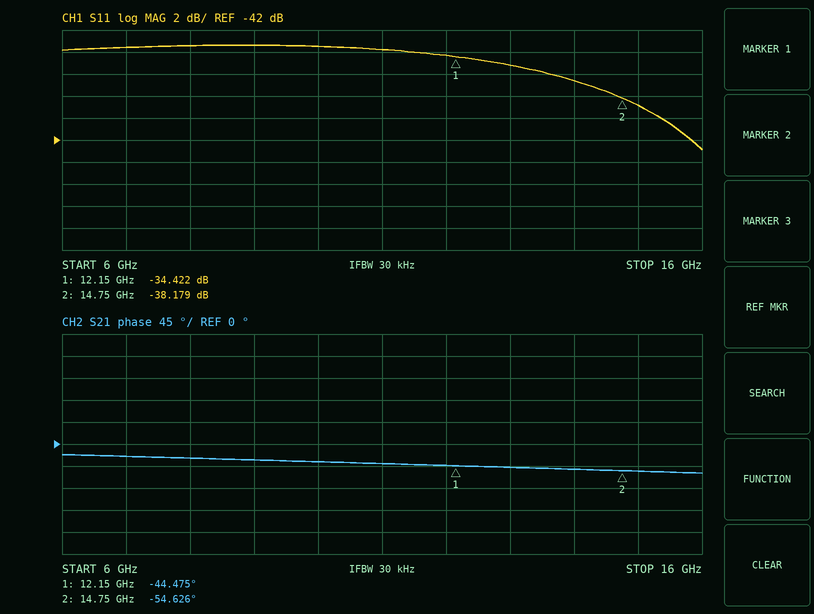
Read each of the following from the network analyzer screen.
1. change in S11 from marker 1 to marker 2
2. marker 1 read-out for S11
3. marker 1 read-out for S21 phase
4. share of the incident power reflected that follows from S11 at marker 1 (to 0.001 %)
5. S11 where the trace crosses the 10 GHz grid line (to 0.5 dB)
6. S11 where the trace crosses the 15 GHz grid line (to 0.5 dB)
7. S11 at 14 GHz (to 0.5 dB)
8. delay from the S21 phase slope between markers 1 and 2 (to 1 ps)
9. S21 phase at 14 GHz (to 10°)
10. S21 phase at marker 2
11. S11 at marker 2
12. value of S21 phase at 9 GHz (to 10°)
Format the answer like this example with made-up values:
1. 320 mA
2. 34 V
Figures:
1. -3.757 dB
2. -34.422 dB
3. -44.475°
4. 0.036 %
5. -33.5 dB
6. -39.0 dB
7. -36.5 dB
8. 11 ps
9. -50°
10. -54.626°
11. -38.179 dB
12. -30°
